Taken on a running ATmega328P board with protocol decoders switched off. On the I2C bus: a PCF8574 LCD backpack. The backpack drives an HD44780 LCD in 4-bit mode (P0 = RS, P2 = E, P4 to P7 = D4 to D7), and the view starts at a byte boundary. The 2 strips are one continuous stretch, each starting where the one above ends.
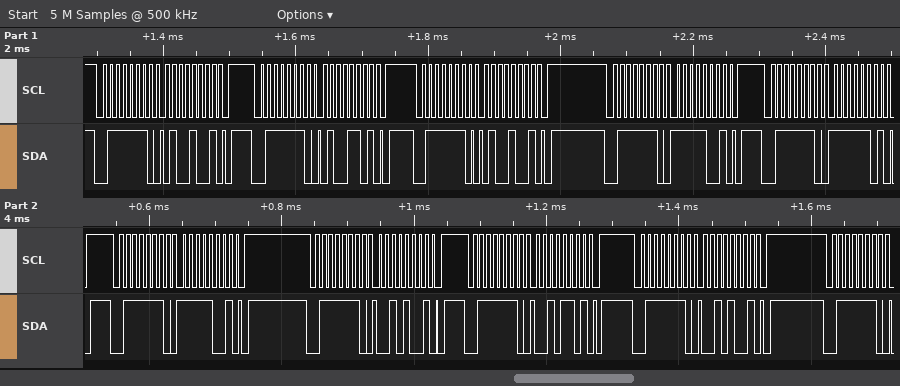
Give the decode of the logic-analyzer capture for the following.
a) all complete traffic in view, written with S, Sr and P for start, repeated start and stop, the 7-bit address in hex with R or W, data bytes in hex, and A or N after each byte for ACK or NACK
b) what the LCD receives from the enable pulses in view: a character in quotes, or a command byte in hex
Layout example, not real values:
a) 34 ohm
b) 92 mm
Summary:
a) S 3FW A 49 A P S 3FW A 4D A P S 3FW A 49 A P S 3FW A F9 A P S 3FW A FD A P S 3FW A F9 A P S 3FW A 29 A P S 3FW A 2D A P S 3FW A 29 A P S 3FW A
b) 'O'
